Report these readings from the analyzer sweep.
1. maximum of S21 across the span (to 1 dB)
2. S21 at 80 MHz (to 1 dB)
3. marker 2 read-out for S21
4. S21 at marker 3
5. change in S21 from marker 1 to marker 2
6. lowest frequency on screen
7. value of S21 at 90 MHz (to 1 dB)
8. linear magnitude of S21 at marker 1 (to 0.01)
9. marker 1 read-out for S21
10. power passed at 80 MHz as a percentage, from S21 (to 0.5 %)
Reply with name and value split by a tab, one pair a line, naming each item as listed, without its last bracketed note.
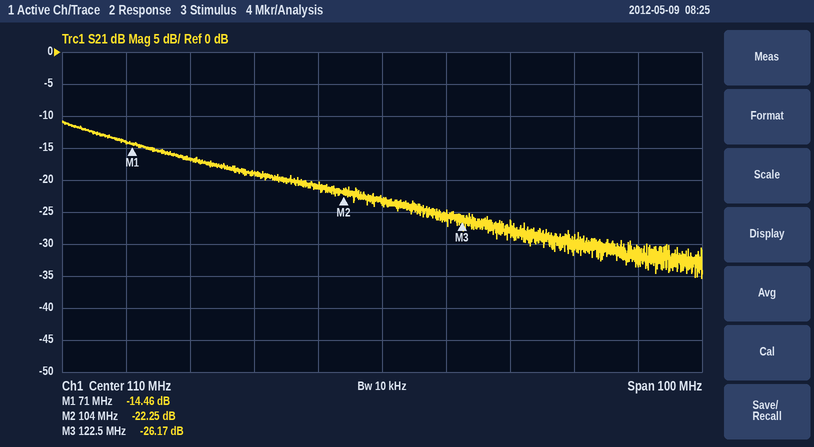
maximum of S21 across the span	-11 dB
S21 at 80 MHz	-17 dB
marker 2 read-out for S21	-22.25 dB
S21 at marker 3	-26.17 dB
change in S21 from marker 1 to marker 2	-7.79 dB
lowest frequency on screen	60 MHz
value of S21 at 90 MHz	-19 dB
linear magnitude of S21 at marker 1	0.19
marker 1 read-out for S21	-14.46 dB
power passed at 80 MHz as a percentage, from S21	2.0 %
